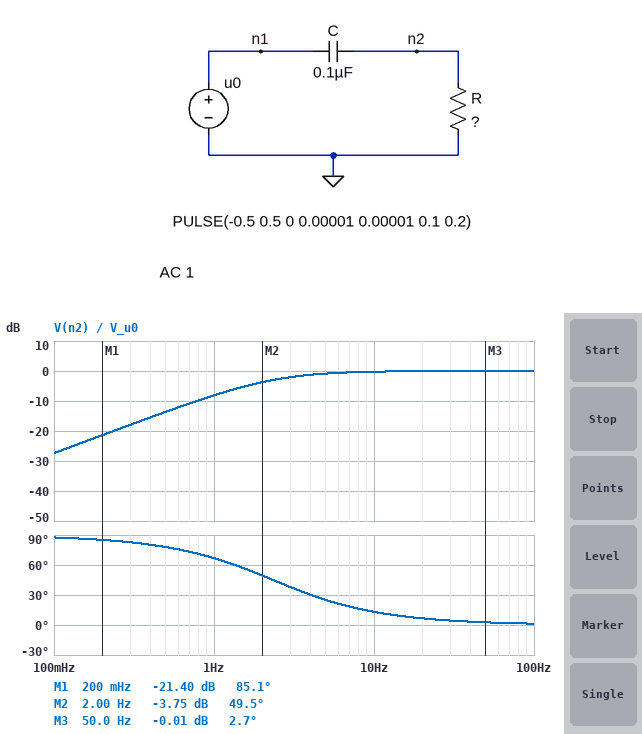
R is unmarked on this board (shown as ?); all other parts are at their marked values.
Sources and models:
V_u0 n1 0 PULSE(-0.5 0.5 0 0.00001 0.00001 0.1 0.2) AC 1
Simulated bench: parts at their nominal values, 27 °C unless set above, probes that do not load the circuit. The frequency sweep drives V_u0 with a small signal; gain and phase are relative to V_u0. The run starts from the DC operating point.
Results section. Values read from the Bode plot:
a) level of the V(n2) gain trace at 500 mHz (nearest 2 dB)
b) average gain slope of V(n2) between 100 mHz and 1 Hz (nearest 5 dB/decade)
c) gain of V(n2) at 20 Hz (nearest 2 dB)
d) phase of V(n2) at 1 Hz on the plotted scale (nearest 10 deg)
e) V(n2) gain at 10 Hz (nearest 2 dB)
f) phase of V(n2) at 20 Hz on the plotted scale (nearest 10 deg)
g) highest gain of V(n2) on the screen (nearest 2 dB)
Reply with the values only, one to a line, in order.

-14 dB
20 dB/decade
0 dB
70 deg
0 dB
10 deg
0 dB
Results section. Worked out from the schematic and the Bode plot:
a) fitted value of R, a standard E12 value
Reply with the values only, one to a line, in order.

680 kΩ
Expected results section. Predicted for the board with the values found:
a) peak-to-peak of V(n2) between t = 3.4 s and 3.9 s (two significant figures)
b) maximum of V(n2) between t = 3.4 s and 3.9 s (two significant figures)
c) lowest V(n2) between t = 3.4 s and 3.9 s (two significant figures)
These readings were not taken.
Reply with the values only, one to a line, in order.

1.6 V
810 mV
-810 mV
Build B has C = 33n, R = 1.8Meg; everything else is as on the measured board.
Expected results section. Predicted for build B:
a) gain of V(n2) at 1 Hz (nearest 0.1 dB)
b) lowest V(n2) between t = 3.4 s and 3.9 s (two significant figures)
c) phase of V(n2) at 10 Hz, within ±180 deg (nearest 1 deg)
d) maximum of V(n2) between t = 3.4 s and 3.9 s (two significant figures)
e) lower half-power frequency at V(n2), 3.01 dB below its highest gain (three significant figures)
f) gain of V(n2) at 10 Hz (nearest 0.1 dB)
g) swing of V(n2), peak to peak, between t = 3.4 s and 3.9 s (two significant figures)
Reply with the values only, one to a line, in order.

-9.1 dB
-840 mV
15 deg
840 mV
2.68 Hz
-0.3 dB
1.7 V
